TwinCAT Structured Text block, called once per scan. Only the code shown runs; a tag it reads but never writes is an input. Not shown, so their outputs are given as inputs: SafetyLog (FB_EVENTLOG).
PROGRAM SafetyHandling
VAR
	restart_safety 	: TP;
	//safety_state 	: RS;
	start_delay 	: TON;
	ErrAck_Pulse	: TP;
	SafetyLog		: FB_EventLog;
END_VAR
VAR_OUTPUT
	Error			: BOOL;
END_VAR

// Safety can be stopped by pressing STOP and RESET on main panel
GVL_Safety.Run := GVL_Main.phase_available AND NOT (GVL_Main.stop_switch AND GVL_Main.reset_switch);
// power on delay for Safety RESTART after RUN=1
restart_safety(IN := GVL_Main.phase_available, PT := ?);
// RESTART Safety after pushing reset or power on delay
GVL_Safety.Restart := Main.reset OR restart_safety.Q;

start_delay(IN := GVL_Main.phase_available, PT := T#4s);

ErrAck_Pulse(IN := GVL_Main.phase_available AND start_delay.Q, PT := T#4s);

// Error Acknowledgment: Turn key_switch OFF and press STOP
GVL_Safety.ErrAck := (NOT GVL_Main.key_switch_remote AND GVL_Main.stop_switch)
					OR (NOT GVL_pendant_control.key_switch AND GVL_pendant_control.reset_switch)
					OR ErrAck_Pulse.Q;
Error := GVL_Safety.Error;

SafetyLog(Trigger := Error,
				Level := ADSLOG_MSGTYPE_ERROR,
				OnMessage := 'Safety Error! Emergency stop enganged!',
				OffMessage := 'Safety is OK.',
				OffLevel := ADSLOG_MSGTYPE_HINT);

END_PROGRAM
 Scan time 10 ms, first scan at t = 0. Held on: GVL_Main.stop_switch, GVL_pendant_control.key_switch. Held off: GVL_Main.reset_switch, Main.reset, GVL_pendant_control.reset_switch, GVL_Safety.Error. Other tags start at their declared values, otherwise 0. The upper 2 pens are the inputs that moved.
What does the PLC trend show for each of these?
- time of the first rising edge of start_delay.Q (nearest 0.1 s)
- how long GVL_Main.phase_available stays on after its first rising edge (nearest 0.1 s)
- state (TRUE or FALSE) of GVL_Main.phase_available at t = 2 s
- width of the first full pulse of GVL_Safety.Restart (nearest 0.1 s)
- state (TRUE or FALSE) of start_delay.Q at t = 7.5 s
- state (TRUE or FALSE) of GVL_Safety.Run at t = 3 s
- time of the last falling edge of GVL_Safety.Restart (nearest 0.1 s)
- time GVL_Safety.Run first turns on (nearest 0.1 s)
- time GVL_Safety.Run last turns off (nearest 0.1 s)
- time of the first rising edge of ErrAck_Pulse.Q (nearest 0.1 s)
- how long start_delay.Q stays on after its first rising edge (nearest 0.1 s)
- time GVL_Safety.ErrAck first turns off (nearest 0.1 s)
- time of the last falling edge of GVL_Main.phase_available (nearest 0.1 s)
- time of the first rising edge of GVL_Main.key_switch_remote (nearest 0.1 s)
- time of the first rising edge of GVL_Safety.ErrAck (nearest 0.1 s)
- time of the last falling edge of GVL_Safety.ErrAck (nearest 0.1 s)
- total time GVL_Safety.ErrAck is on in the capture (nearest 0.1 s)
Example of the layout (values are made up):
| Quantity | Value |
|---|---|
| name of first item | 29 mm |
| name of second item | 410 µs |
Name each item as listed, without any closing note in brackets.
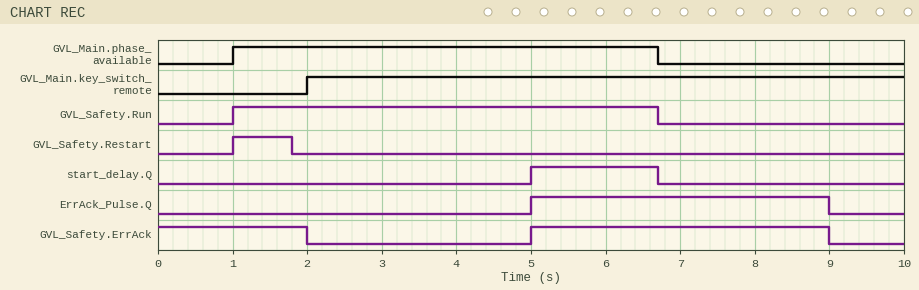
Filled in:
| Quantity | Value |
|---|---|
| time of the first rising edge of start_delay.Q | 5.0 s |
| how long GVL_Main.phase_available stays on after its first rising edge | 5.7 s |
| state (TRUE or FALSE) of GVL_Main.phase_available at t = 2 s | TRUE |
| width of the first full pulse of GVL_Safety.Restart | 0.8 s |
| state (TRUE or FALSE) of start_delay.Q at t = 7.5 s | FALSE |
| state (TRUE or FALSE) of GVL_Safety.Run at t = 3 s | TRUE |
| time of the last falling edge of GVL_Safety.Restart | 1.8 s |
| time GVL_Safety.Run first turns on | 1.0 s |
| time GVL_Safety.Run last turns off | 6.7 s |
| time of the first rising edge of ErrAck_Pulse.Q | 5.0 s |
| how long start_delay.Q stays on after its first rising edge | 1.7 s |
| time GVL_Safety.ErrAck first turns off | 2.0 s |
| time of the last falling edge of GVL_Main.phase_available | 6.7 s |
| time of the first rising edge of GVL_Main.key_switch_remote | 2.0 s |
| time of the first rising edge of GVL_Safety.ErrAck | 5.0 s |
| time of the last falling edge of GVL_Safety.ErrAck | 9.0 s |
| total time GVL_Safety.ErrAck is on in the capture | 6.0 s |
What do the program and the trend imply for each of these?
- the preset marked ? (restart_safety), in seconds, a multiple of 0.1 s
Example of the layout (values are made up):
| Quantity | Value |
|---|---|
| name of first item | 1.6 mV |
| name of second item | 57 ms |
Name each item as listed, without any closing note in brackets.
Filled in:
| Quantity | Value |
|---|---|
| the preset marked ? (restart_safety), in seconds, a multiple of 0.1 s | 0.8 s |
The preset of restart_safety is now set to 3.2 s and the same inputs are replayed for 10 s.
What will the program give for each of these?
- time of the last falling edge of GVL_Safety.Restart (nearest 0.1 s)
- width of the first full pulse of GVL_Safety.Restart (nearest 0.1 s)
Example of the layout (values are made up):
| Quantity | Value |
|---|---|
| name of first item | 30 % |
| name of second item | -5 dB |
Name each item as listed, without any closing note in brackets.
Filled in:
| Quantity | Value |
|---|---|
| time of the last falling edge of GVL_Safety.Restart | 4.2 s |
| width of the first full pulse of GVL_Safety.Restart | 3.2 s |
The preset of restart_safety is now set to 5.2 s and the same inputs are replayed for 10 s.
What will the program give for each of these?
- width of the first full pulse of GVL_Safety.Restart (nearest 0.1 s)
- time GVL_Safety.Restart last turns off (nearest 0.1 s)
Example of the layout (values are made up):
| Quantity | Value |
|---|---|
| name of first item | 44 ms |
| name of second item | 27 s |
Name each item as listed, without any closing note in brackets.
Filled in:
| Quantity | Value |
|---|---|
| width of the first full pulse of GVL_Safety.Restart | 5.2 s |
| time GVL_Safety.Restart last turns off | 6.2 s |
